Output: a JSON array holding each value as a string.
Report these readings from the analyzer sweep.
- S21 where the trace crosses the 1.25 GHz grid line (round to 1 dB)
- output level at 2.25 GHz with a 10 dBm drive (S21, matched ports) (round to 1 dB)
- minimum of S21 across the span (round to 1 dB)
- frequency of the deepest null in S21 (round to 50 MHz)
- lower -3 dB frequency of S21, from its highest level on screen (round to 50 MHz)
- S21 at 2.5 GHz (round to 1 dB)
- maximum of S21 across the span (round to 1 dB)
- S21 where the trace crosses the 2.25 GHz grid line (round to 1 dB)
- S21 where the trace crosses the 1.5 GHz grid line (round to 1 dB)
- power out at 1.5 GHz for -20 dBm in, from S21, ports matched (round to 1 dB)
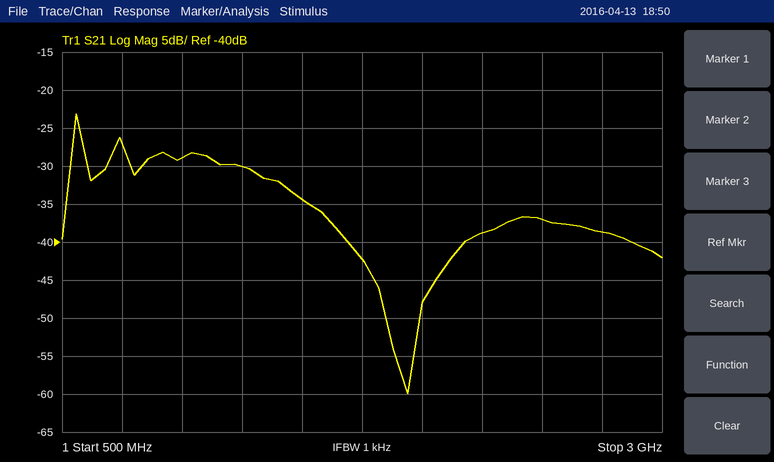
["-30 dB", "-29 dBm", "-60 dB", "1.95 GHz", "550 MHz", "-37 dB", "-23 dB", "-39 dB", "-34 dB", "-54 dBm"]
